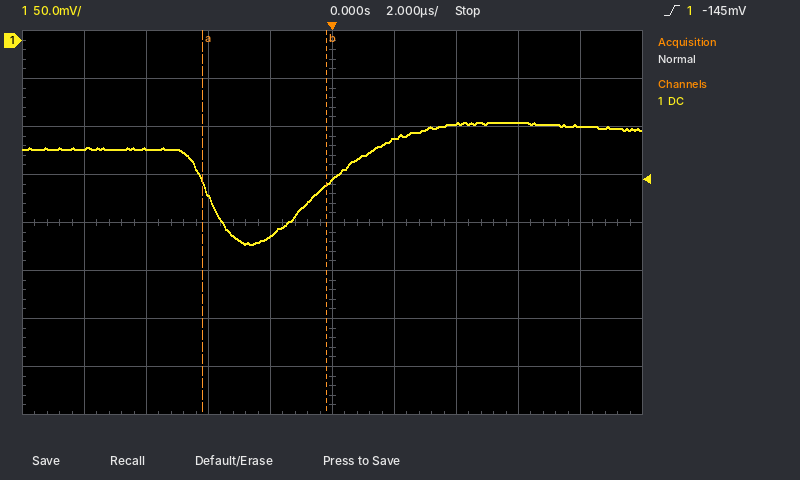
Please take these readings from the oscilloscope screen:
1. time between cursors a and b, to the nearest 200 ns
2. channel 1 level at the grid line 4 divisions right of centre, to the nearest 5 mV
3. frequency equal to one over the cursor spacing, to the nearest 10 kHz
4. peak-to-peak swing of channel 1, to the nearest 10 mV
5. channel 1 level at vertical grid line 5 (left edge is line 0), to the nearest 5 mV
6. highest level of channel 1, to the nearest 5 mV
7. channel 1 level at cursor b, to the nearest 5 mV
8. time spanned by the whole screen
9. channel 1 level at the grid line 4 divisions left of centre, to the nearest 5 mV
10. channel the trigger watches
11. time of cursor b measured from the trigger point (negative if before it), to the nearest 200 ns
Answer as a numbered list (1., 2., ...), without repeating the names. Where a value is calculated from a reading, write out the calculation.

1. 4.0 µs
2. -90 mV
3. 1 / 4.0 µs ≈ 250 kHz
4. 130 mV
5. -145 mV
6. -85 mV
7. -150 mV
8. 20 µs
9. -115 mV
10. channel 1
11. -200 ns
